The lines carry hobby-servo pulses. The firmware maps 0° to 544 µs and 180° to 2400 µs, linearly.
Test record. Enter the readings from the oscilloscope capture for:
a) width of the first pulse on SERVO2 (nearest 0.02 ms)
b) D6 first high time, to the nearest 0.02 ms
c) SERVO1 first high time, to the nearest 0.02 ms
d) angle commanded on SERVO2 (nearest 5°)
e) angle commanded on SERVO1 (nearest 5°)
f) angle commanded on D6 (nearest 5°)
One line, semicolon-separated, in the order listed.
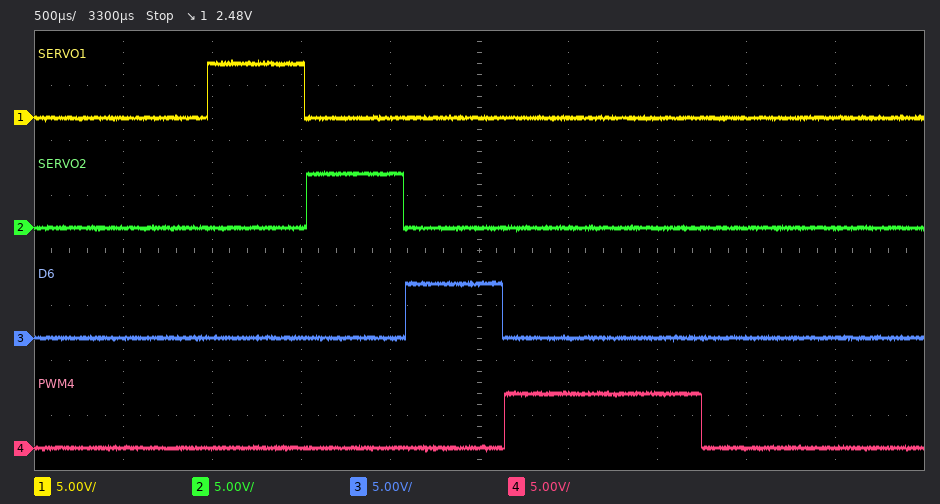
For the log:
0.54 ms; 0.54 ms; 0.54 ms; 0°; 0°; 0°
